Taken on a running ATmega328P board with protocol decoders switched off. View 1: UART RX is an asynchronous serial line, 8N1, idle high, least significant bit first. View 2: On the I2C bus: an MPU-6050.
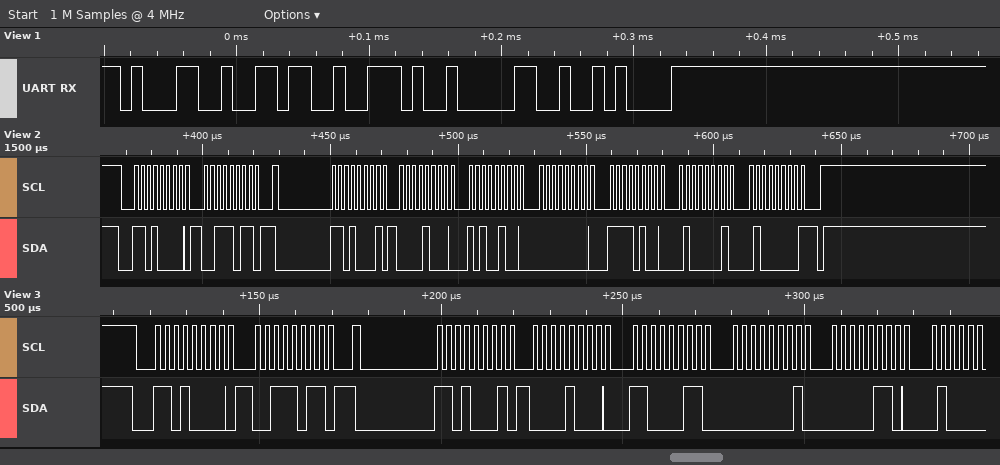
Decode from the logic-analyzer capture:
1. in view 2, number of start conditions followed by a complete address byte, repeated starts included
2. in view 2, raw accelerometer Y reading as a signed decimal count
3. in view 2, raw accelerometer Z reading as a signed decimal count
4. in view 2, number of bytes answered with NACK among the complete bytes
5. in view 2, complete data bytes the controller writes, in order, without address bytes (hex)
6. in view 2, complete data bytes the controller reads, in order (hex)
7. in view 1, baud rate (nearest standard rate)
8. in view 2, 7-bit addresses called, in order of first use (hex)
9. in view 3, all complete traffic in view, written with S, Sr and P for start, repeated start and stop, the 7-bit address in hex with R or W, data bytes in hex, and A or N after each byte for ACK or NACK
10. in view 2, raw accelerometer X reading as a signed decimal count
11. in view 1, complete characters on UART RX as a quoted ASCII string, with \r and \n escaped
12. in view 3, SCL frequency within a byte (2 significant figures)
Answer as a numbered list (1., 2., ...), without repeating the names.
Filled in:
1. 2
2. 244
3. 16704
4. 1
5. 3B
6. 08 A4 00 F4 41 40
7. 115200 baud
8. 0x68
9. S 68W A 3B A Sr 68R A 08 A C3 A 01 A 06 A
10. 2212
11. "16.0\n"
12. 400 kHz
